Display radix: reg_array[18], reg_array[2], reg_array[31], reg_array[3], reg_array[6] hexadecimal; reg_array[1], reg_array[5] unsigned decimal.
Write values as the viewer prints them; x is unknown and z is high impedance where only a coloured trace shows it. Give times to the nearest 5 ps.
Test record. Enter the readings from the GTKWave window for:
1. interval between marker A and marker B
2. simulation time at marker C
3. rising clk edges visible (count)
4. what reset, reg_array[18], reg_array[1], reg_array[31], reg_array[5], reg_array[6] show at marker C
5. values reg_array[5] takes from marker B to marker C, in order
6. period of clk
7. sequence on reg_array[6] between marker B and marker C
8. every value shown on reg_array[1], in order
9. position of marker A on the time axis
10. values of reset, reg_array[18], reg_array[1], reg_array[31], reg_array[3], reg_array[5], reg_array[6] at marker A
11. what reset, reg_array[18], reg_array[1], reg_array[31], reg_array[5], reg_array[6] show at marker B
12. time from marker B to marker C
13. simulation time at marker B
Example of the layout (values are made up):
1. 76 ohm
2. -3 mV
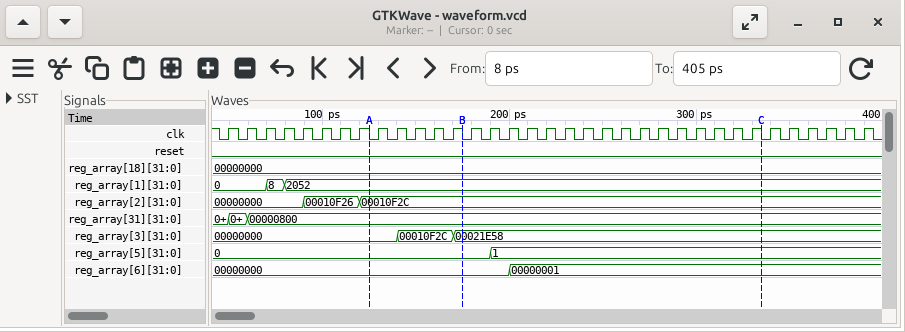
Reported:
1. 50 ps
2. 335 ps
3. 35
4. reset=0, reg_array[18]=00000000, reg_array[1]=2052, reg_array[31]=00000800, reg_array[5]=1, reg_array[6]=00000001
5. 0, 1
6. 10 ps
7. 00000000, 00000001
8. 0, 8, 2052
9. 125 ps
10. reset=0, reg_array[18]=00000000, reg_array[1]=2052, reg_array[31]=00000800, reg_array[3]=00000000, reg_array[5]=0, reg_array[6]=00000000
11. reset=0, reg_array[18]=00000000, reg_array[1]=2052, reg_array[31]=00000800, reg_array[5]=0, reg_array[6]=00000000
12. 160 ps
13. 175 ps
